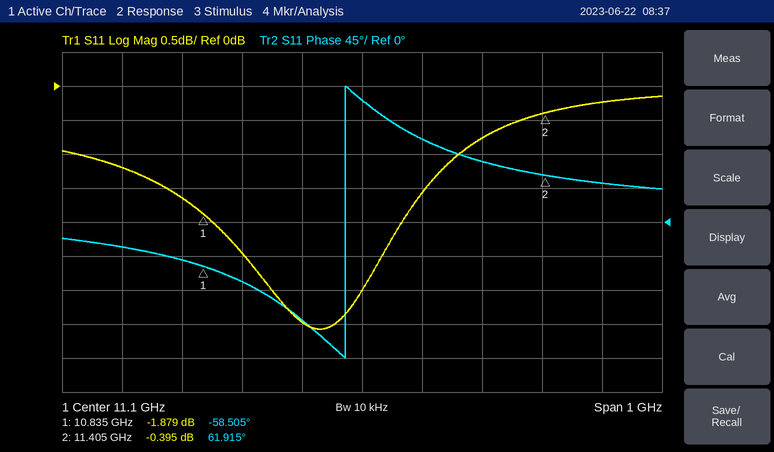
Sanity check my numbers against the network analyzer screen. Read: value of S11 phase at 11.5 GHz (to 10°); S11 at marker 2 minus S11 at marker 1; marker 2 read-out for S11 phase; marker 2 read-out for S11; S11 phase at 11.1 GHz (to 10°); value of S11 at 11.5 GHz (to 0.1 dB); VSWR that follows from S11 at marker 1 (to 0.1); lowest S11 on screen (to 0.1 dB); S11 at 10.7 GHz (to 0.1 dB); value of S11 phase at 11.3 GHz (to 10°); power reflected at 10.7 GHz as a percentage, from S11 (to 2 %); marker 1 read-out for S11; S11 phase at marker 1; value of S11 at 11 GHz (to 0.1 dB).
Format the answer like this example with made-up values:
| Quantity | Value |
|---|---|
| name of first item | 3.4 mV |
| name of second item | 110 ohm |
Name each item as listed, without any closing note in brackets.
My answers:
| Quantity | Value |
|---|---|
| value of S11 phase at 11.5 GHz | 50° |
| S11 at marker 2 minus S11 at marker 1 | 1.484 dB |
| marker 2 read-out for S11 phase | 61.915° |
| marker 2 read-out for S11 | -0.395 dB |
| S11 phase at 11.1 GHz | 160° |
| value of S11 at 11.5 GHz | -0.2 dB |
| VSWR that follows from S11 at marker 1 | 9.3 |
| lowest S11 on screen | -3.6 dB |
| S11 at 10.7 GHz | -1.2 dB |
| value of S11 phase at 11.3 GHz | 80° |
| power reflected at 10.7 GHz as a percentage, from S11 | 76 % |
| marker 1 read-out for S11 | -1.879 dB |
| S11 phase at marker 1 | -58.505° |
| value of S11 at 11 GHz | -3.5 dB |
